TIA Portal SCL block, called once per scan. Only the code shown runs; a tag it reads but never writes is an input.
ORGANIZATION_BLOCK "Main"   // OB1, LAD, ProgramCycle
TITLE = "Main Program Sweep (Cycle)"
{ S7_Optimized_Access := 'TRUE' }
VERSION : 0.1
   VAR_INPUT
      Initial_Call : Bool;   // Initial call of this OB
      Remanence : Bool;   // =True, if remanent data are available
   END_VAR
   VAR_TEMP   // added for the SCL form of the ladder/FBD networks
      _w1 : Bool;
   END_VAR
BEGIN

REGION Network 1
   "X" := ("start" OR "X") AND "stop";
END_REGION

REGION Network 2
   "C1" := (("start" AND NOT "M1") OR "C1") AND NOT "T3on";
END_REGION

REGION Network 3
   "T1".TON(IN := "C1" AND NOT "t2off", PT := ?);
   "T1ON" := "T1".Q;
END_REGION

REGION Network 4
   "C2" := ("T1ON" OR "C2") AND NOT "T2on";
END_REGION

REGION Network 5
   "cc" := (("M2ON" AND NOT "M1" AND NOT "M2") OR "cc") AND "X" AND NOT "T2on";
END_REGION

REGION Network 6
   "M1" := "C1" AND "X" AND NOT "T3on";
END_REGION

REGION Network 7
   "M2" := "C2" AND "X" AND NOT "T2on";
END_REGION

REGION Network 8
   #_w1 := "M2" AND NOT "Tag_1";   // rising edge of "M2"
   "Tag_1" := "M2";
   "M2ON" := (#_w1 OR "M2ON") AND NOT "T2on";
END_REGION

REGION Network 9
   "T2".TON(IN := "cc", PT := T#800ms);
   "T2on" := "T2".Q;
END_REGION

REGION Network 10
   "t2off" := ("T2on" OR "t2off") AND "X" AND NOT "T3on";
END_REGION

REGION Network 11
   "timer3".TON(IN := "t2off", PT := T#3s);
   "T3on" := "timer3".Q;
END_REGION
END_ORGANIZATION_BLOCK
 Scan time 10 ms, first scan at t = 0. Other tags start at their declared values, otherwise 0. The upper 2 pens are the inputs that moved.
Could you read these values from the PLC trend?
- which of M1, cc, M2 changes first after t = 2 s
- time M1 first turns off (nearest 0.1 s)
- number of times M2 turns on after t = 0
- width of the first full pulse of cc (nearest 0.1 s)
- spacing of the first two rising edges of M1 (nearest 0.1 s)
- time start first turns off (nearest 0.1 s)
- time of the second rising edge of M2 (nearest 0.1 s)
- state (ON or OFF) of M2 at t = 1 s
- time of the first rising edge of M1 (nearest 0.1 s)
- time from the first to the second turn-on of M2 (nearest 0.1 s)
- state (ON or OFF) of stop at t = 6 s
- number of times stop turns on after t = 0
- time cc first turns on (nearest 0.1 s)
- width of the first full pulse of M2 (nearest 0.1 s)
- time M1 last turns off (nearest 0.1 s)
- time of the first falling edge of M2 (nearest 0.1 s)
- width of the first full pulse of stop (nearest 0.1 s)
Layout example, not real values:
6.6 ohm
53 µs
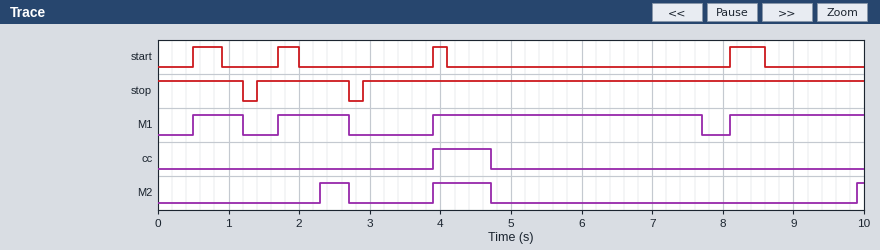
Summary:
M2
1.2 s
3
0.8 s
1.2 s
0.9 s
3.9 s
OFF
0.5 s
1.6 s
ON
2
3.9 s
0.4 s
7.7 s
2.7 s
1.3 s
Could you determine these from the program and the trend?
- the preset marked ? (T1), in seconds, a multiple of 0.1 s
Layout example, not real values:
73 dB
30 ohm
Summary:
1.8 s
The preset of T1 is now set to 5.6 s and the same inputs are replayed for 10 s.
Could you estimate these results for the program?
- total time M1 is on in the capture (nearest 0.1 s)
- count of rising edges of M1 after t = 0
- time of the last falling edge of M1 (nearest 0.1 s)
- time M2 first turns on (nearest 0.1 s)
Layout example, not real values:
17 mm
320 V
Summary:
7.8 s
3
2.7 s
6.1 s
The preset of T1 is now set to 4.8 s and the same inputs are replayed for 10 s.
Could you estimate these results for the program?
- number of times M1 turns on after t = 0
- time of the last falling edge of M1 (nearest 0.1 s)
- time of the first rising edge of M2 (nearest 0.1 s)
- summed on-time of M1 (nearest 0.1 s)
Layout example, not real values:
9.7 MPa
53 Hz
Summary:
3
2.7 s
5.3 s
7.8 s
